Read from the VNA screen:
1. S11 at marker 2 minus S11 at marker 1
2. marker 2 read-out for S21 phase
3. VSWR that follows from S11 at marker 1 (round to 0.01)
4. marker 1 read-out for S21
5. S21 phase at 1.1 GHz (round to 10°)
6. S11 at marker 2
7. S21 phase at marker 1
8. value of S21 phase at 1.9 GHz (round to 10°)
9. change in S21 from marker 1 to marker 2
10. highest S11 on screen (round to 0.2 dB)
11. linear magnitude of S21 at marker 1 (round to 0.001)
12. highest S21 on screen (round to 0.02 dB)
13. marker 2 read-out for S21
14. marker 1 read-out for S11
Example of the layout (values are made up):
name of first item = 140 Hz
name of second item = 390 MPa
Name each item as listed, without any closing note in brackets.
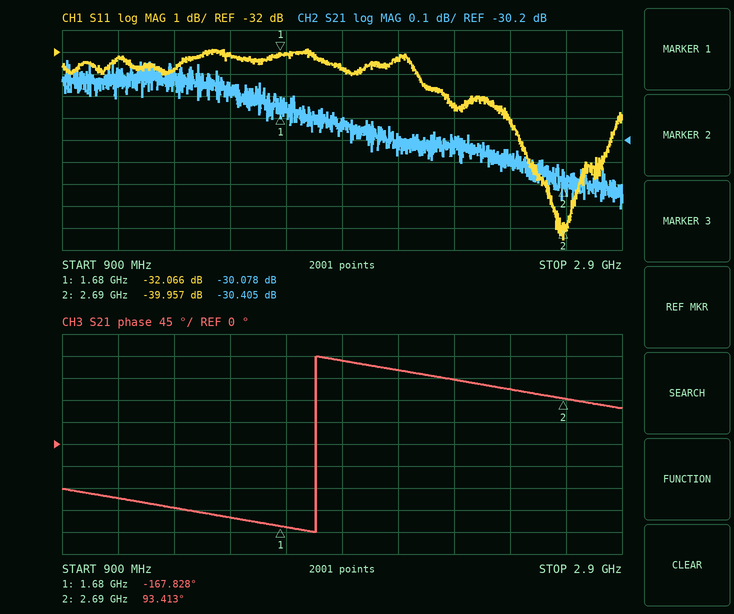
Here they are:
S11 at marker 2 minus S11 at marker 1 = -7.891 dB
marker 2 read-out for S21 phase = 93.413°
VSWR that follows from S11 at marker 1 = 1.05
marker 1 read-out for S21 = -30.078 dB
S21 phase at 1.1 GHz = -110°
S11 at marker 2 = -39.957 dB
S21 phase at marker 1 = -167.828°
value of S21 phase at 1.9 GHz = 170°
change in S21 from marker 1 to marker 2 = -0.327 dB
highest S11 on screen = -31.8 dB
linear magnitude of S21 at marker 1 = 0.031
highest S21 on screen = -29.84 dB
marker 2 read-out for S21 = -30.405 dB
marker 1 read-out for S11 = -32.066 dB
